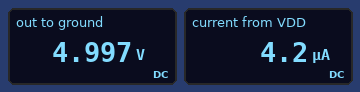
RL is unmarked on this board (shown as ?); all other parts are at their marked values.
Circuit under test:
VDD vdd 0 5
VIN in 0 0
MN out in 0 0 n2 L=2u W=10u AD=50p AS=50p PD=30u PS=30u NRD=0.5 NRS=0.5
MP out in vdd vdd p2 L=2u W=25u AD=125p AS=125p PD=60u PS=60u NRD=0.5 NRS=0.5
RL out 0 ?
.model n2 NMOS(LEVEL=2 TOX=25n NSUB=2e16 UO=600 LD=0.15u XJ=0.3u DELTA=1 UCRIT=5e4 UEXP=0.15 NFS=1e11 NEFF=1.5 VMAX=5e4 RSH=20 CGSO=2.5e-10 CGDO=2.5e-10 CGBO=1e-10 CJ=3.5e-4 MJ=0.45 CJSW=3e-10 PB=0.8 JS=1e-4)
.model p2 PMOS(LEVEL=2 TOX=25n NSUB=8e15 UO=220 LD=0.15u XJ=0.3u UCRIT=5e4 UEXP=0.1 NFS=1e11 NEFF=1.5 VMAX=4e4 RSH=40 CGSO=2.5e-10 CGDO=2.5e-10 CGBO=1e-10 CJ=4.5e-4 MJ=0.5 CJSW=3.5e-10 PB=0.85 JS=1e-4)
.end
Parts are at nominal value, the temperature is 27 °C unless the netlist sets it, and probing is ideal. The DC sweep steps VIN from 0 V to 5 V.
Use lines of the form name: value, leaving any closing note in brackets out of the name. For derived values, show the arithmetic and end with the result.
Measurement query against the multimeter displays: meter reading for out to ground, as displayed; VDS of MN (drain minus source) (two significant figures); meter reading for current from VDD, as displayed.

meter reading for out to ground, as displayed: 4.997 V
VDS of MN (drain minus source): 4.997 V = 5.0 V
meter reading for current from VDD, as displayed: 4.2 µA
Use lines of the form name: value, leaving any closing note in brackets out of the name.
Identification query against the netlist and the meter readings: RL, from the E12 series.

RL, from the E12 series: 1.2 MΩ
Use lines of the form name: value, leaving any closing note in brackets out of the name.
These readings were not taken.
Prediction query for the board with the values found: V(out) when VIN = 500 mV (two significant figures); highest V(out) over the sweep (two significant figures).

V(out) when VIN = 500 mV: 5.0 V
highest V(out) over the sweep: 5.0 V
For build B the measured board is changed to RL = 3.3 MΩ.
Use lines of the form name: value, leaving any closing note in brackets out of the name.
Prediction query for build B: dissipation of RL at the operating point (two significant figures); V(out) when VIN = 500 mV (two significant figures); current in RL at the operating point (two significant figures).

dissipation of RL at the operating point: 7.6 µW
V(out) when VIN = 500 mV: 5.0 V
current in RL at the operating point: 1.5 µA
